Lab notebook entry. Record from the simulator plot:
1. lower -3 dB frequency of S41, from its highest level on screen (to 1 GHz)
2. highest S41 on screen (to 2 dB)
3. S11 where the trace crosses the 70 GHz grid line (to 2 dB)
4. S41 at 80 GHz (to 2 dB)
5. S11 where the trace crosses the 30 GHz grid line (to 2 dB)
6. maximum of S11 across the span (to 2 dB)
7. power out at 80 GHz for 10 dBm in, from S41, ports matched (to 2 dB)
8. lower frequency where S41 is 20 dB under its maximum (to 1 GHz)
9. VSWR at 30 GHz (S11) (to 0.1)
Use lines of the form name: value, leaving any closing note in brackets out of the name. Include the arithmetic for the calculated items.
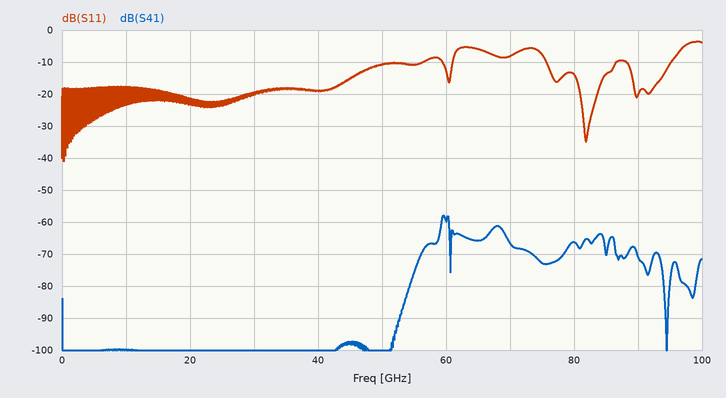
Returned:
lower -3 dB frequency of S41, from its highest level on screen: 59 GHz
highest S41 on screen: -58 dB
S11 where the trace crosses the 70 GHz grid line: -8 dB
S41 at 80 GHz: -66 dB
S11 where the trace crosses the 30 GHz grid line: -20 dB
maximum of S11 across the span: -4 dB
power out at 80 GHz for 10 dBm in, from S41, ports matched: 10 dBm + (-66 dB) = -56 dBm
lower frequency where S41 is 20 dB under its maximum: 55 GHz
VSWR at 30 GHz (S11): |Γ| = 10^(-20/20) = 0.1000; VSWR = (1 + 0.1000)/(1 − 0.1000) ≈ 1.2
